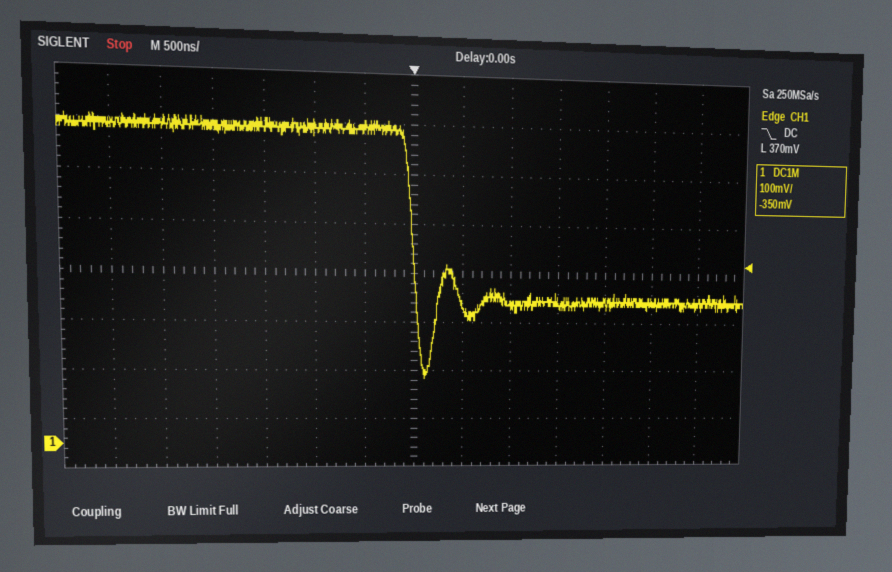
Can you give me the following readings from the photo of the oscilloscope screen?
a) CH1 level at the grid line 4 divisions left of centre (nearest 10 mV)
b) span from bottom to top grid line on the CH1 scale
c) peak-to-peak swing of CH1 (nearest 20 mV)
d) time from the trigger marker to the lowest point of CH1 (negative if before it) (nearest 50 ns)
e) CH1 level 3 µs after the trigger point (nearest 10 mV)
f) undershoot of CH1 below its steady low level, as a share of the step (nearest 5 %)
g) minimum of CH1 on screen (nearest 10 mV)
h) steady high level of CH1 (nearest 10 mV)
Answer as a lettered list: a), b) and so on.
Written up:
a) 640 mV
b) 800 mV
c) 520 mV
d) +100 ns
e) 290 mV
f) 45 %
g) 140 mV
h) 640 mV
